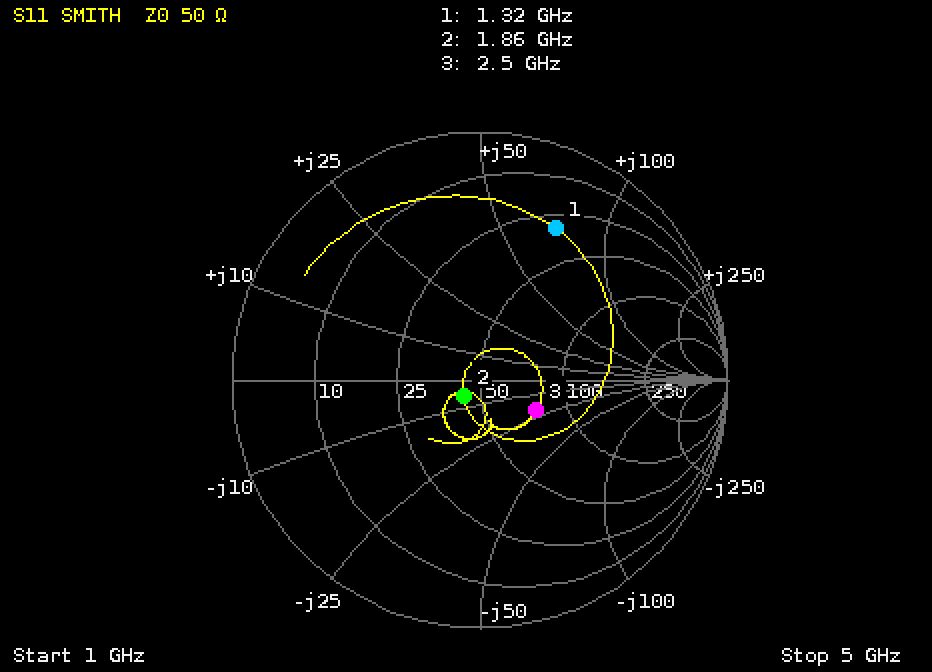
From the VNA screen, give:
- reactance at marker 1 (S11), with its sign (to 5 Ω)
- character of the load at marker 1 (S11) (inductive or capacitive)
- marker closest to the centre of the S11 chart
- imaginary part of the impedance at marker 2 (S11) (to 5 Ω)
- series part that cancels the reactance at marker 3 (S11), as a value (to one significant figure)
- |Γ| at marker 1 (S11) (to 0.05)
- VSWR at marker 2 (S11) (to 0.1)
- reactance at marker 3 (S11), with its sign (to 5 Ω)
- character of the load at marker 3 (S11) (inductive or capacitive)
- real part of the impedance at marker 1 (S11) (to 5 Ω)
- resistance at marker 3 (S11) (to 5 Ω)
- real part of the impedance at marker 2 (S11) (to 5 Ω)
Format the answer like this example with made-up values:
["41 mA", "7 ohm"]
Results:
["+70 Ω", "inductive", "marker 2", "-5 Ω", "1 nH", "0.70", "1.2", "-20 Ω", "capacitive", "30 Ω", "75 Ω", "45 Ω"]
